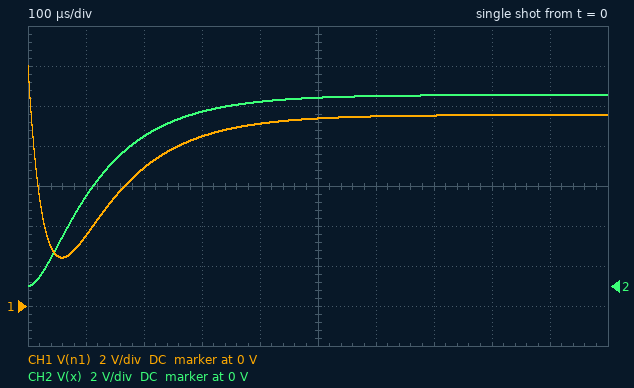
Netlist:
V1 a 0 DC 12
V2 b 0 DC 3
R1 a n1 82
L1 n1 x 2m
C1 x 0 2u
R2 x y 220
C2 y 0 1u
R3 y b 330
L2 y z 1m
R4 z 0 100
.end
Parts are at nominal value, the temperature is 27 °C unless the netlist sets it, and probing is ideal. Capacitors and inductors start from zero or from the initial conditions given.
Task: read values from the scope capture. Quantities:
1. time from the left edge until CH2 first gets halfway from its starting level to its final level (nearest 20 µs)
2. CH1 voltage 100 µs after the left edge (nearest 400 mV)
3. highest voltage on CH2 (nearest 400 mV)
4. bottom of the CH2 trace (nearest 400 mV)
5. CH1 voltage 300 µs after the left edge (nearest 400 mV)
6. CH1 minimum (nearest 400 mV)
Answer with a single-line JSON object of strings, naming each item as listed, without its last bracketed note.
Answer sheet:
{"time from the left edge until CH2 first gets halfway from its starting level to its final level": "100 µs", "CH1 voltage 100 µs after the left edge": "3.6 V", "highest voltage on CH2": "9.6 V", "bottom of the CH2 trace": "0 V", "CH1 voltage 300 µs after the left edge": "8.4 V", "CH1 minimum": "2.4 V"}
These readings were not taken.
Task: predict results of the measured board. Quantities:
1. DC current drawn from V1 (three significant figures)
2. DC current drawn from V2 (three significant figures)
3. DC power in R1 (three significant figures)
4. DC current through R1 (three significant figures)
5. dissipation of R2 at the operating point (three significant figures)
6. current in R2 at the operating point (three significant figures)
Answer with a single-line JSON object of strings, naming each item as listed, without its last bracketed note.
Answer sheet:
{"DC current drawn from V1": "29.8 mA", "DC current drawn from V2": "36.8 µA", "DC power in R1": "73.0 mW", "DC current through R1": "29.8 mA", "dissipation of R2 at the operating point": "196 mW", "current in R2 at the operating point": "29.8 mA"}
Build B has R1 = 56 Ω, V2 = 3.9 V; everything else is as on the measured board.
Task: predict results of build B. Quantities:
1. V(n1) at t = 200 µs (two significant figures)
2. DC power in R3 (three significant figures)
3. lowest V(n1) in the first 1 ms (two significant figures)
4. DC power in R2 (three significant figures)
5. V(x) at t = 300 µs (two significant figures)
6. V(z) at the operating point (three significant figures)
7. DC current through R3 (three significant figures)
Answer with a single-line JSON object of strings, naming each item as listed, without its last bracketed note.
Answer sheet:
{"V(n1) at t = 200 µs": "8.3 V", "DC power in R3": "1.02 mW", "lowest V(n1) in the first 1 ms": "3.5 V", "DC power in R2": "218 mW", "V(x) at t = 300 µs": "10 V", "V(z) at the operating point": "3.32 V", "DC current through R3": "1.76 mA"}
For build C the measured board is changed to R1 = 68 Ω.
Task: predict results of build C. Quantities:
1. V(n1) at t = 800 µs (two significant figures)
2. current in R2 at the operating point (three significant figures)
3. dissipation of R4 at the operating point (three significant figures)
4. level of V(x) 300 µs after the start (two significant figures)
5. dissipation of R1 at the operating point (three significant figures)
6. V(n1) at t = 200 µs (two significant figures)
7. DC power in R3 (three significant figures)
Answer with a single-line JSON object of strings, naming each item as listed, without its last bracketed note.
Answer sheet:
{"V(n1) at t = 800 µs": "9.9 V", "current in R2 at the operating point": "31.0 mA", "dissipation of R4 at the operating point": "94.6 mW", "level of V(x) 300 µs after the start": "9.4 V", "dissipation of R1 at the operating point": "65.3 mW", "V(n1) at t = 200 µs": "7.6 V", "DC power in R3": "17.4 µW"}
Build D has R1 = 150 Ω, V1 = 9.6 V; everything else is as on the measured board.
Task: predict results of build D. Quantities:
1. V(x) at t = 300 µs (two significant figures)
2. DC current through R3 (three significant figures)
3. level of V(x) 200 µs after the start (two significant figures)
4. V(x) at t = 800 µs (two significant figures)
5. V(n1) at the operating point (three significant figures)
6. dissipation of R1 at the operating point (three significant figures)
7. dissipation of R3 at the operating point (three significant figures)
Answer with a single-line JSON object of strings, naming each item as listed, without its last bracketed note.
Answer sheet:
{"V(x) at t = 300 µs": "5.1 V", "DC current through R3": "2.34 mA", "level of V(x) 200 µs after the start": "4.0 V", "V(x) at t = 800 µs": "6.5 V", "V(n1) at the operating point": "6.61 V", "dissipation of R1 at the operating point": "59.6 mW", "dissipation of R3 at the operating point": "1.81 mW"}
